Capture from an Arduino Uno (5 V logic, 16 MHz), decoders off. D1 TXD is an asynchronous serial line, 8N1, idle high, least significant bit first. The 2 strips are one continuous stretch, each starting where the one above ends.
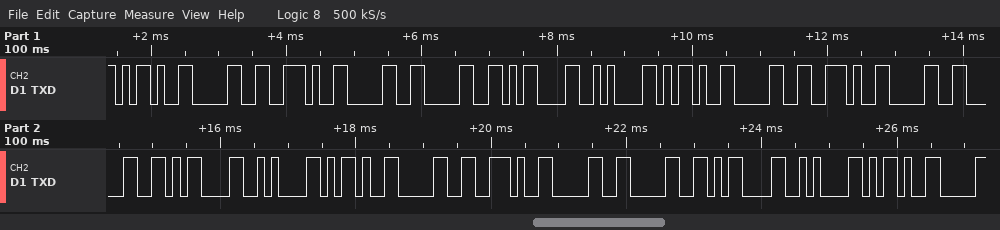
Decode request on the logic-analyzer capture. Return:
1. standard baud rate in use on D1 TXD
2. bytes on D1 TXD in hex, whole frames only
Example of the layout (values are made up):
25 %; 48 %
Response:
9600 baud; 0x2D 0x30 0x2E 0x30 0x30 0x0D 0x0A 0x2D 0x30 0x2E 0x30 0x30 0x0D 0x0A 0x2D 0x30 0x2E 0x30 0x30 0x0D 0x0A 0x2D
